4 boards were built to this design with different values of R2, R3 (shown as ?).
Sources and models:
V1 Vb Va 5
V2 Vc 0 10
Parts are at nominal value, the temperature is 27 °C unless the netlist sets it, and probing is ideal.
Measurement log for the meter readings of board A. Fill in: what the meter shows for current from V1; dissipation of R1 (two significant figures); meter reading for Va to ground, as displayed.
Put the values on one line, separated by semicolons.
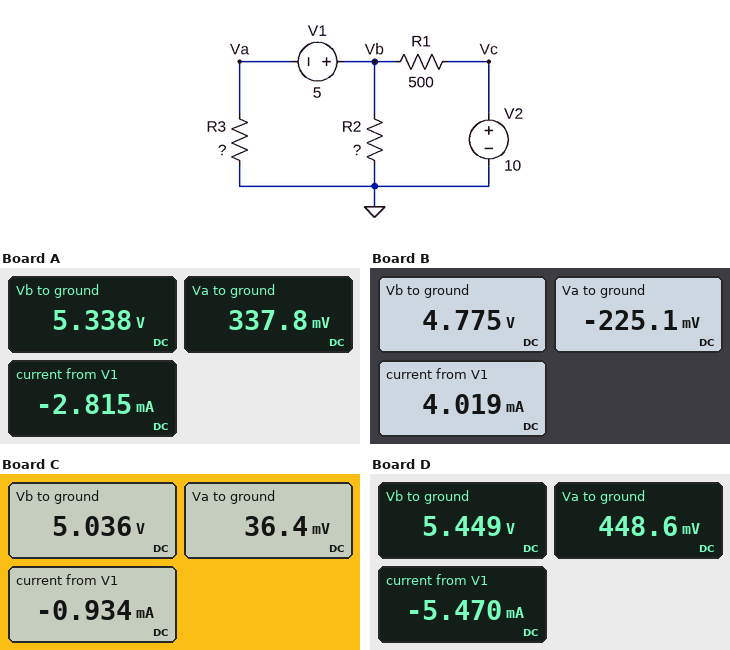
-2.815 mA; 43 mW; 337.8 mV
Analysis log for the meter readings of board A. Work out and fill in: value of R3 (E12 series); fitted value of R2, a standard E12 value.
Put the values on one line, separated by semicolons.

120 Ω; 820 Ω
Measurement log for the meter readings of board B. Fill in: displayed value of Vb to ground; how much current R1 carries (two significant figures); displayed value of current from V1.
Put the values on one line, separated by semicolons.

4.775 V; 10 mA; 4.019 mA
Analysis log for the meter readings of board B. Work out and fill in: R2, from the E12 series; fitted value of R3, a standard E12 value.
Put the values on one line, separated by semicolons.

330 Ω; 56 Ω
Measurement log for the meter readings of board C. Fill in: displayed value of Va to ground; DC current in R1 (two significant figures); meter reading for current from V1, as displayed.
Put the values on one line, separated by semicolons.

36.4 mV; 9.9 mA; -0.934 mA
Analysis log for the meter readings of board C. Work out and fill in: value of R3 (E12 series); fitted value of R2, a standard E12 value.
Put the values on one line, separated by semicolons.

39 Ω; 560 Ω
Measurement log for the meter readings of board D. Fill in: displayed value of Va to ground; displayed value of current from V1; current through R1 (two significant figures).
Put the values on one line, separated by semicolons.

448.6 mV; -5.470 mA; 9.1 mA
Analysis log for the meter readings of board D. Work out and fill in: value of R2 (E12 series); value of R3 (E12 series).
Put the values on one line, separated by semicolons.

1.5 kΩ; 82 Ω
